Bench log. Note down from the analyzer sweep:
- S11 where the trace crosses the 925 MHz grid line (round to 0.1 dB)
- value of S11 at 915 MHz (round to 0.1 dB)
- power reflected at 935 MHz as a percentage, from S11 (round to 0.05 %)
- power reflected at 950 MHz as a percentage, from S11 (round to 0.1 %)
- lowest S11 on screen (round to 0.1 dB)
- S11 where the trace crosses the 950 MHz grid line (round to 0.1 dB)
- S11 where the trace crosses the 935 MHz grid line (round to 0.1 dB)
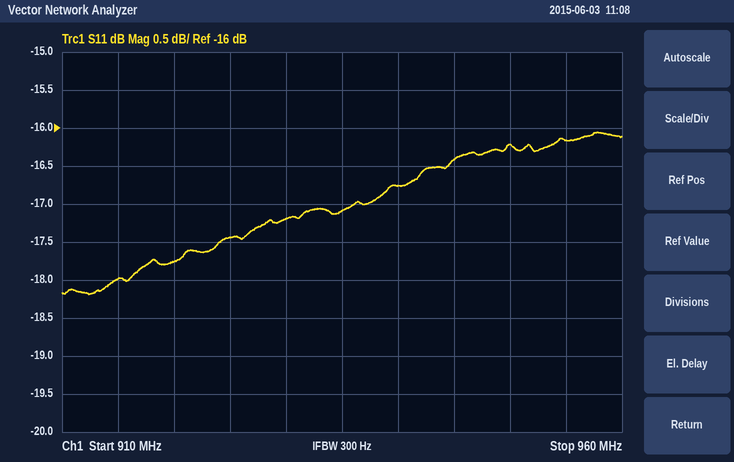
-17.4 dB
-18.0 dB
1.95 %
2.4 %
-18.2 dB
-16.2 dB
-17.1 dB
